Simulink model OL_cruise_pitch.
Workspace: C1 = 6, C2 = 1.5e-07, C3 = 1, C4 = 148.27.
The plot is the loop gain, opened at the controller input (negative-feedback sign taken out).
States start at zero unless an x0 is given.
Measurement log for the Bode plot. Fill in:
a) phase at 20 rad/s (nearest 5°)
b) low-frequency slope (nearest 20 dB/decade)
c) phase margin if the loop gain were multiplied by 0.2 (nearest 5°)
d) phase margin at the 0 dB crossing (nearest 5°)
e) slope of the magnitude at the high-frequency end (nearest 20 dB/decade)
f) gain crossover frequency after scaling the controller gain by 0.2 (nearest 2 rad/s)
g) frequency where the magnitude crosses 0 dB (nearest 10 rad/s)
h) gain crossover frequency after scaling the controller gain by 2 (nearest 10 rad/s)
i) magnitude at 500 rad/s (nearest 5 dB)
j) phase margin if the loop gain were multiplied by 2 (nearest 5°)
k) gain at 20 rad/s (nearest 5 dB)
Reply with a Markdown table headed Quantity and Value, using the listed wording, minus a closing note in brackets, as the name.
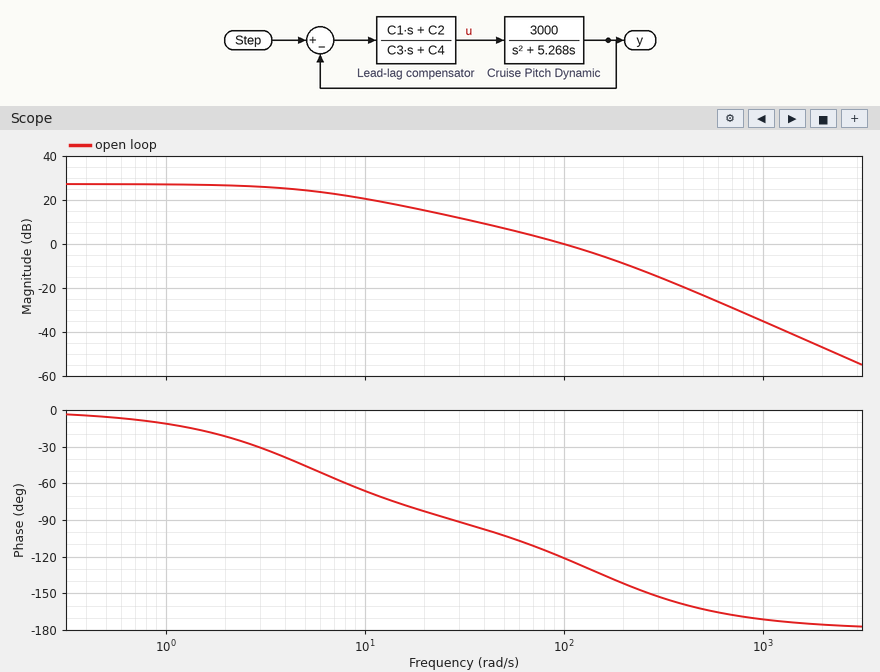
| Quantity | Value |
|---|---|
| phase at 20 rad/s | -85° |
| low-frequency slope | 0 dB/decade |
| phase margin if the loop gain were multiplied by 0.2 | 95° |
| phase margin at the 0 dB crossing | 60° |
| slope of the magnitude at the high-frequency end | -40 dB/decade |
| gain crossover frequency after scaling the controller gain by 0.2 | 24 rad/s |
| frequency where the magnitude crosses 0 dB | 100 rad/s |
| gain crossover frequency after scaling the controller gain by 2 | 160 rad/s |
| magnitude at 500 rad/s | -25 dB |
| phase margin if the loop gain were multiplied by 2 | 45° |
| gain at 20 rad/s | 15 dB |
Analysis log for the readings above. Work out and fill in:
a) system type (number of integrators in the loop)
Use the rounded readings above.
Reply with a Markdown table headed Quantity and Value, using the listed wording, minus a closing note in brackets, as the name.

| Quantity | Value |
|---|---|
| system type | 0 |
